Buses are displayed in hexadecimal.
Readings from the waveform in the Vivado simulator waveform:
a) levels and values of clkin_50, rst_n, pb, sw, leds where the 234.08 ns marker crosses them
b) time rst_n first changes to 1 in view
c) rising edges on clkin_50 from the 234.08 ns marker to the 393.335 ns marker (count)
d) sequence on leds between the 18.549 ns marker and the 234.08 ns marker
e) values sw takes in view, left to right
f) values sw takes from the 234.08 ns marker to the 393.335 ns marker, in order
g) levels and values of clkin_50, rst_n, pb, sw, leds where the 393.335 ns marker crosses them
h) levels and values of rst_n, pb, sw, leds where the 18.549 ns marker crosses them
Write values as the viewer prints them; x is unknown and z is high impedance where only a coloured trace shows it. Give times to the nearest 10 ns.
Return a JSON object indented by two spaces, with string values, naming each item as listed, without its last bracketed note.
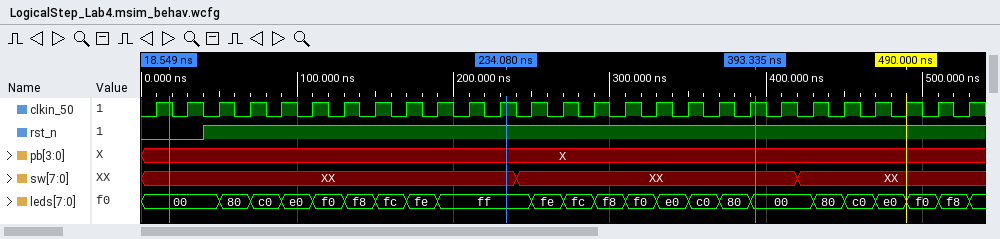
{
  "levels and values of clkin_50, rst_n, pb, sw, leds where the 234.08 ns marker crosses them": "clkin_50=1, rst_n=1, pb=X, sw=XX, leds=ff",
  "time rst_n first changes to 1 in view": "40 ns",
  "rising edges on clkin_50 from the 234.08 ns marker to the 393.335 ns marker": "8",
  "sequence on leds between the 18.549 ns marker and the 234.08 ns marker": "00, 80, c0, e0, f0, f8, fc, fe, ff",
  "values sw takes in view, left to right": "XX, XX, XX",
  "values sw takes from the 234.08 ns marker to the 393.335 ns marker, in order": "XX, XX",
  "levels and values of clkin_50, rst_n, pb, sw, leds where the 393.335 ns marker crosses them": "clkin_50=1, rst_n=1, pb=X, sw=XX, leds=00",
  "levels and values of rst_n, pb, sw, leds where the 18.549 ns marker crosses them": "rst_n=0, pb=X, sw=XX, leds=00"
}
